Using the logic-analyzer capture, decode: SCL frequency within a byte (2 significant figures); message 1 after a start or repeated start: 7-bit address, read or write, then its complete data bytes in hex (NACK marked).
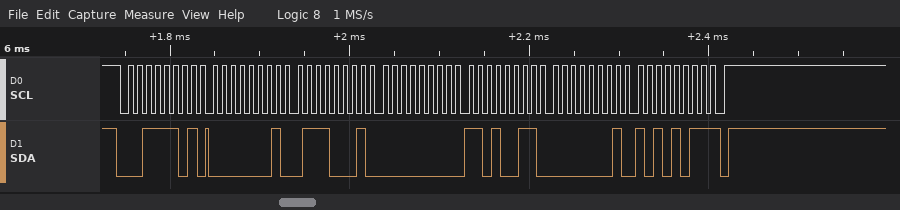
100 kHz
0x1E read: 01 71 00 D3 01 AB NACK
